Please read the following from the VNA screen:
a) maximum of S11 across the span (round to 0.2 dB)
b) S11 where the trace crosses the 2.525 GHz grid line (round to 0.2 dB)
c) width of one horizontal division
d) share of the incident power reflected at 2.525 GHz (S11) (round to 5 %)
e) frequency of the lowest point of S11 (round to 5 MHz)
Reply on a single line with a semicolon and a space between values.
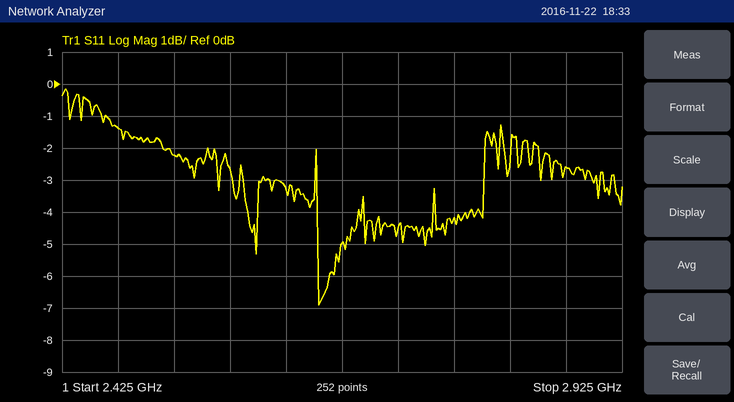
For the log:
-0.2 dB; -2.2 dB; 50 MHz; 60 %; 2.655 GHz
